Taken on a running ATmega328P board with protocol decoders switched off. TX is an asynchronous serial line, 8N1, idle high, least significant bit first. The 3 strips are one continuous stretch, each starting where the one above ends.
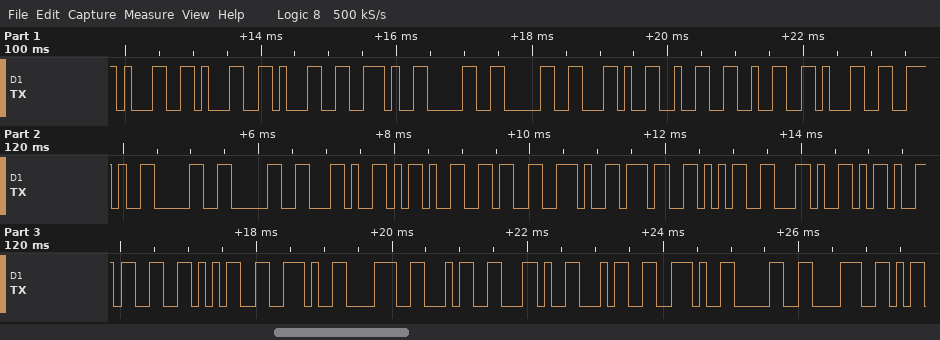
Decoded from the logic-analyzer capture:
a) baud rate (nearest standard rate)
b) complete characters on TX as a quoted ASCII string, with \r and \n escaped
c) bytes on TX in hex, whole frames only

9600 baud
"111.00,221.00,-6.75,-35.84,4.08"
0x31 0x31 0x31 0x2E 0x30 0x30 0x2C 0x32 0x32 0x31 0x2E 0x30 0x30 0x2C 0x2D 0x36 0x2E 0x37 0x35 0x2C 0x2D 0x33 0x35 0x2E 0x38 0x34 0x2C 0x34 0x2E 0x30 0x38
